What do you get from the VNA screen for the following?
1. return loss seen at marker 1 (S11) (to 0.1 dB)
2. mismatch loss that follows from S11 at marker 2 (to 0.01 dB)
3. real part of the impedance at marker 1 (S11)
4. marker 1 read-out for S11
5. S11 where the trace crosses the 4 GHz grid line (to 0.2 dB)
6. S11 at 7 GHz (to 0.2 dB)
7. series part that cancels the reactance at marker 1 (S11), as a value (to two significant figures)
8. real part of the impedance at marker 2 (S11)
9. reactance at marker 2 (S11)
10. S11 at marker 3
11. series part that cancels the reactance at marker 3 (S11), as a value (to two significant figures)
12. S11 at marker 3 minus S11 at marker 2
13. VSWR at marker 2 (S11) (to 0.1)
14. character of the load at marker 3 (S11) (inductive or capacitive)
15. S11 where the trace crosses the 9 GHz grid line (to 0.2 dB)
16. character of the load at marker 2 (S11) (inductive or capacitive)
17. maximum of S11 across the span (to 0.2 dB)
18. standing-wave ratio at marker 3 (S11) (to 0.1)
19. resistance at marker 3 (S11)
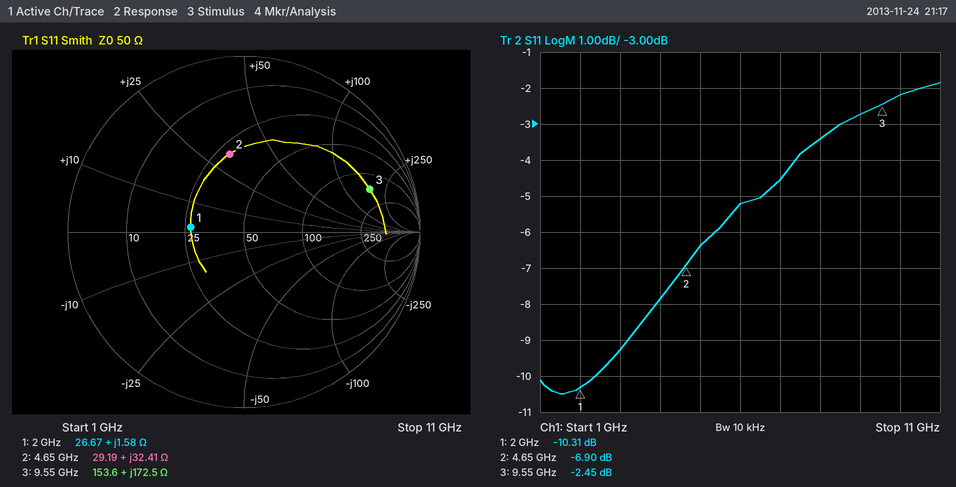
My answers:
10.3 dB
0.99 dB
26.67 Ω
-10.31 dB
-7.8 dB
-4.6 dB
50 pF
29.19 Ω
+32.41 Ω
-2.45 dB
97 fF
4.45 dB
2.6
inductive
-2.8 dB
inductive
-1.8 dB
7.1
153.6 Ω
